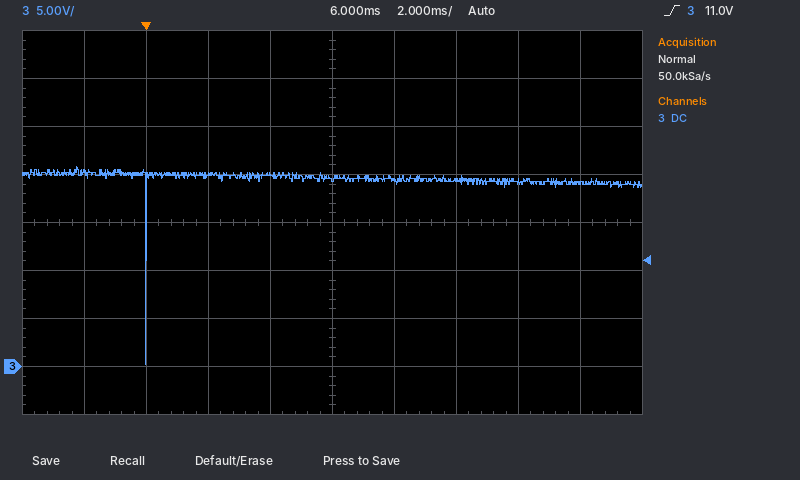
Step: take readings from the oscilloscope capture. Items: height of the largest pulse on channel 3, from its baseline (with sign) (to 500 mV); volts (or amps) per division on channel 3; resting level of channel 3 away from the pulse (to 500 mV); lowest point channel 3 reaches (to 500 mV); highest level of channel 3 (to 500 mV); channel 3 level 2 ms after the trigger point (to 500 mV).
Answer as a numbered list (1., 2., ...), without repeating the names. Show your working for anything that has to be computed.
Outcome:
1. 0.0 V − (19.5 V) = -19.5 V
2. 5 V
3. 19.5 V
4. 0.0 V
5. 21.0 V
6. 20.0 V
